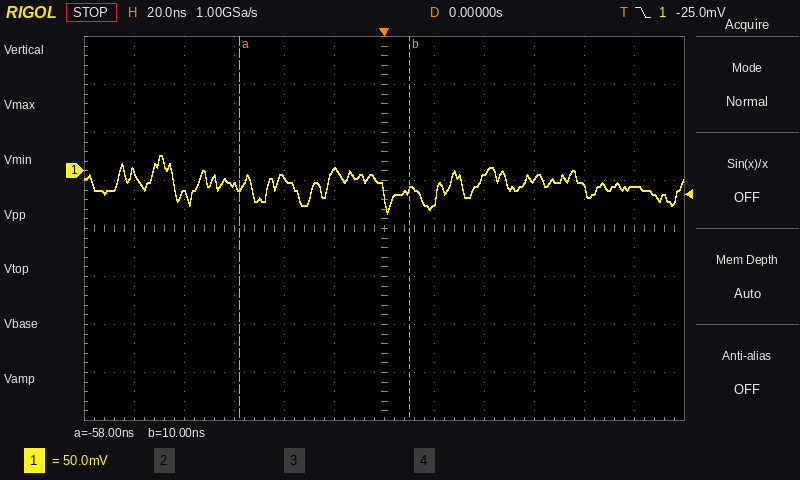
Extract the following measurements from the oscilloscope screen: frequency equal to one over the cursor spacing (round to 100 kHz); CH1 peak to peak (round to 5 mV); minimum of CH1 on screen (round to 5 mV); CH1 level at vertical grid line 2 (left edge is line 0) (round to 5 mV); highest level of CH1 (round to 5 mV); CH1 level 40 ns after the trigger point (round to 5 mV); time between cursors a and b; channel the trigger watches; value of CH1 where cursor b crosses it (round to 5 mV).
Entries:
14.7 MHz
60 mV
-45 mV
-25 mV
15 mV
-5 mV
68 ns
CH1
-20 mV
